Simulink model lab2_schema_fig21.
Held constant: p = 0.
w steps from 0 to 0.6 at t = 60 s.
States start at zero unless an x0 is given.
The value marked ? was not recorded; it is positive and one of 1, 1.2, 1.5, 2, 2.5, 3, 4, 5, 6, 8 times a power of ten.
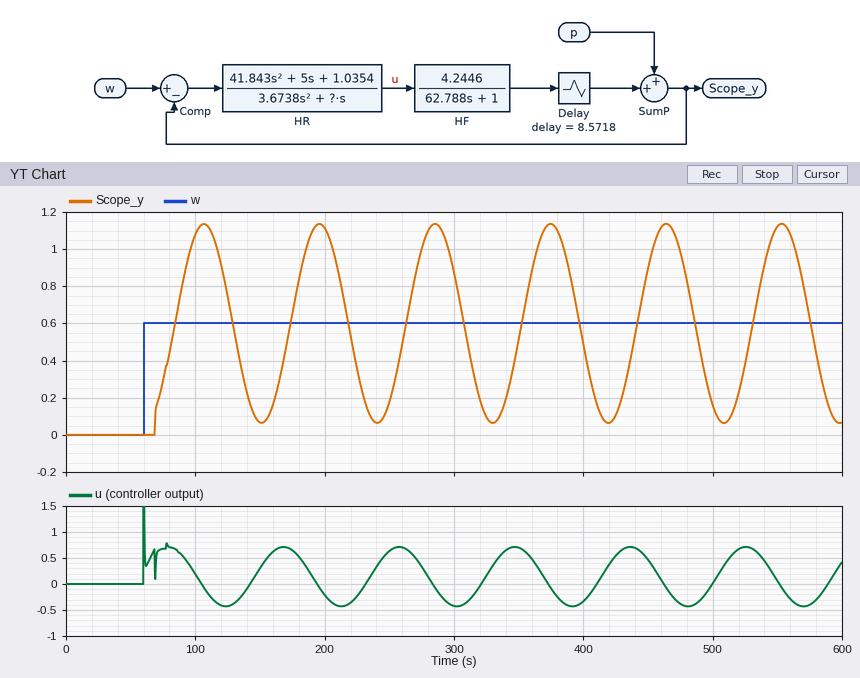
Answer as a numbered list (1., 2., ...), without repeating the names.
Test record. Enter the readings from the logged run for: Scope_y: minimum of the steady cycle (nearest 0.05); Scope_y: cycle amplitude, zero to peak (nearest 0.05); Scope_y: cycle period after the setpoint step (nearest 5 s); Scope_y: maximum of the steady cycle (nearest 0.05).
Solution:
1. 0.05
2. 0.55
3. 90 s
4. 1.15
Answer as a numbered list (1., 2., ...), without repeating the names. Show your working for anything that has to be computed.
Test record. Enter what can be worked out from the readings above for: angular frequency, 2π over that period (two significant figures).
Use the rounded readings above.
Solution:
1. 2π / 90 = 0.070 rad/s
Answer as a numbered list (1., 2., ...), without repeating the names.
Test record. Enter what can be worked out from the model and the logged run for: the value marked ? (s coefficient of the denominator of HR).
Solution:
1. 12
